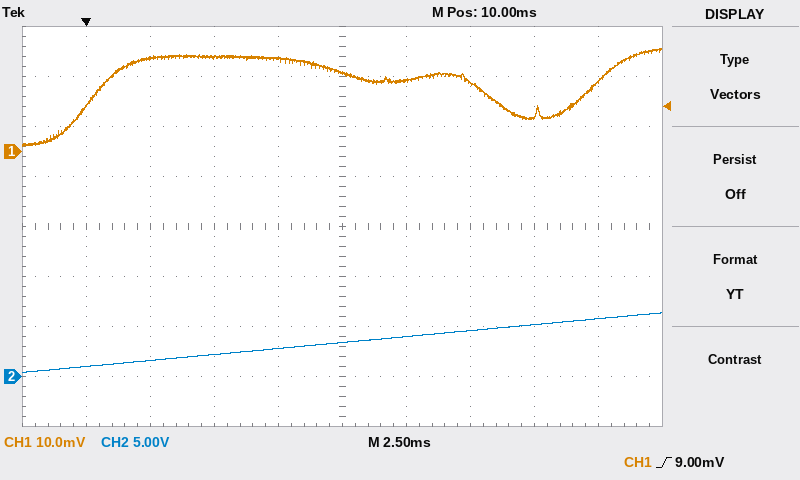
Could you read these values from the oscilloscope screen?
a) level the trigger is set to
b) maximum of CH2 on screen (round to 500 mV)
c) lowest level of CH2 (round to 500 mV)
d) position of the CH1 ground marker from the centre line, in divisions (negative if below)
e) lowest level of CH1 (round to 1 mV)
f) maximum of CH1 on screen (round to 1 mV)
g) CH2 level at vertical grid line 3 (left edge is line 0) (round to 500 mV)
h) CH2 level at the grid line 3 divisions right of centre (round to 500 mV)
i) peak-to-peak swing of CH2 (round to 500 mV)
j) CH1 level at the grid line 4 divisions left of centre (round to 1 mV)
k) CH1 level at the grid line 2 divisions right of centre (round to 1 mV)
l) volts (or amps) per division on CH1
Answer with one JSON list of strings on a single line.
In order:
["9.00 mV", "6.5 V", "500 mV", "+1.5 div", "1 mV", "21 mV", "2.0 V", "5.0 V", "6.0 V", "9 mV", "14 mV", "10 mV"]
